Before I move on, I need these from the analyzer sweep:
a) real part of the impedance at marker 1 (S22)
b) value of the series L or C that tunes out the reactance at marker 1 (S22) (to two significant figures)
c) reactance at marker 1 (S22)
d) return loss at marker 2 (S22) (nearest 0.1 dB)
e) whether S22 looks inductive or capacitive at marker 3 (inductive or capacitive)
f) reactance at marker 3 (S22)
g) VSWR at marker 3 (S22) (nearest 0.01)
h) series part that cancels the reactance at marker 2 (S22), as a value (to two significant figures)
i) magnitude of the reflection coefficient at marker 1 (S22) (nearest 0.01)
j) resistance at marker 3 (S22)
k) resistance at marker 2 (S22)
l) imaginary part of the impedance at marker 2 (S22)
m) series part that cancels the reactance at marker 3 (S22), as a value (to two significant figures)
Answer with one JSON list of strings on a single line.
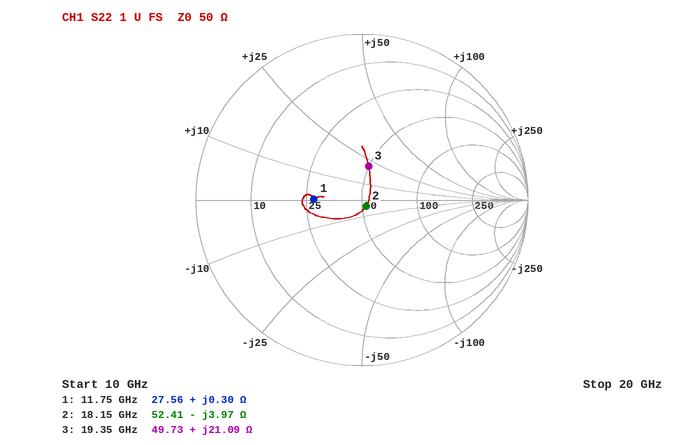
["27.56 Ω", "45 pF", "+0.30 Ω", "26.9 dB", "inductive", "+21.09 Ω", "1.52", "35 pH", "0.29", "49.73 Ω", "52.41 Ω", "-3.97 Ω", "390 fF"]
